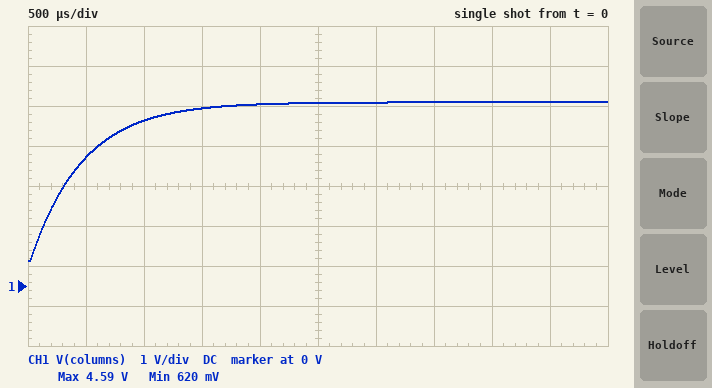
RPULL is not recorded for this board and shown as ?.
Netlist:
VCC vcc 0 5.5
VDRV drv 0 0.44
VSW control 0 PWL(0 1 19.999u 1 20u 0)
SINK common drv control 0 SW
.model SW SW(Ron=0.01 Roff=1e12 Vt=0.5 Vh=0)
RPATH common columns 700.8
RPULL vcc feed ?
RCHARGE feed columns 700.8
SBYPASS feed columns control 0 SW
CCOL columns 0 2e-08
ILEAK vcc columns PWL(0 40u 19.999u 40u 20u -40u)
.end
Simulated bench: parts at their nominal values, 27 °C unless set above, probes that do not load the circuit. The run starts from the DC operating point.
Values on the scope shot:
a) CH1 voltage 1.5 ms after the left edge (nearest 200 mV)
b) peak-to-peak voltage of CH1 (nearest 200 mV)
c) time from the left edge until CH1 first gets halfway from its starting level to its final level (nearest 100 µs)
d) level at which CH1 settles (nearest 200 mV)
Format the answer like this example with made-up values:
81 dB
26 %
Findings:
4.4 V
4.0 V
300 µs
4.6 V
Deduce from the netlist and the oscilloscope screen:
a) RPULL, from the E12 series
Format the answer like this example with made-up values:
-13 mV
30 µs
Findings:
22 kΩ
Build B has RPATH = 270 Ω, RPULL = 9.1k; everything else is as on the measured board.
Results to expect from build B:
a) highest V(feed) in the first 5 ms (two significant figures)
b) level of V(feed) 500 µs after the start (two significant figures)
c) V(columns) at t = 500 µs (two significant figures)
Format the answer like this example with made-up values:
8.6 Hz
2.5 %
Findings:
5.1 V
4.8 V
4.7 V
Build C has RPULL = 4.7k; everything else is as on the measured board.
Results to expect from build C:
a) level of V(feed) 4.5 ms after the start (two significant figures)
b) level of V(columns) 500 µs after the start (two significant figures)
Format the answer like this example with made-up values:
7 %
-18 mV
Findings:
5.3 V
5.2 V
